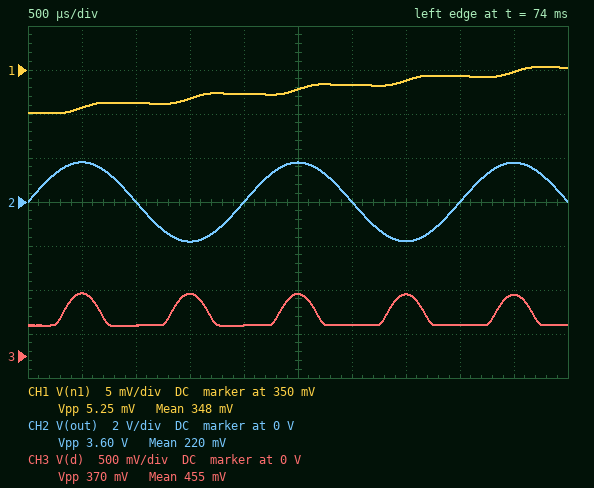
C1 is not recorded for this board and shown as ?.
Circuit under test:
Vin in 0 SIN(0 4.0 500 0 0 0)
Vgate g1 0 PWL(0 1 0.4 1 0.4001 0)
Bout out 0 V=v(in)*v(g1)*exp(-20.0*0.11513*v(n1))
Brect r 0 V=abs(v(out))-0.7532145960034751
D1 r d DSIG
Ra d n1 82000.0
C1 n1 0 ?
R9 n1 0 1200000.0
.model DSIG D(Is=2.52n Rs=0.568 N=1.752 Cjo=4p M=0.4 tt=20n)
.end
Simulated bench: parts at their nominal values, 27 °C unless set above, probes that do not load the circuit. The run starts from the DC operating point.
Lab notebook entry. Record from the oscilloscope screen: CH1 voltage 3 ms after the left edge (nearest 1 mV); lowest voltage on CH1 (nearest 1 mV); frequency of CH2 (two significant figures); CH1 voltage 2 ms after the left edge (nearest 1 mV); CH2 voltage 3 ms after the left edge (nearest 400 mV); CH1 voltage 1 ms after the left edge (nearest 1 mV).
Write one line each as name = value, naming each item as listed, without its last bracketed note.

CH1 voltage 3 ms after the left edge = 348 mV
lowest voltage on CH1 = 345 mV
frequency of CH2 = 500 Hz
CH1 voltage 2 ms after the left edge = 347 mV
CH2 voltage 3 ms after the left edge = 0 V
CH1 voltage 1 ms after the left edge = 346 mV
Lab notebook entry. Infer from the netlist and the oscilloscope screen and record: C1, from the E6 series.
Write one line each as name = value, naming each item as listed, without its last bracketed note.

C1, from the E6 series = 1 µF
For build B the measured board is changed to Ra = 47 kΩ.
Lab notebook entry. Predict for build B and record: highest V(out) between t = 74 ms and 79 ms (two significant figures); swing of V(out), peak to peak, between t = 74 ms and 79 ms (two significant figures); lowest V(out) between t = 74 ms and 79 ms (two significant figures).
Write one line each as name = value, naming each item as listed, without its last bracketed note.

highest V(out) between t = 74 ms and 79 ms = 1.7 V
swing of V(out), peak to peak, between t = 74 ms and 79 ms = 3.3 V
lowest V(out) between t = 74 ms and 79 ms = -1.7 V
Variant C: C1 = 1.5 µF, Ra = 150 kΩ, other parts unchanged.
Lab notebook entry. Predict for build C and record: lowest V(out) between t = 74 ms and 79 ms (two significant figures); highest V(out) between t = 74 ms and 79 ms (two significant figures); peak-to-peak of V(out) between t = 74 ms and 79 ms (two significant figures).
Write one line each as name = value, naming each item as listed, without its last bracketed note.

lowest V(out) between t = 74 ms and 79 ms = -2.3 V
highest V(out) between t = 74 ms and 79 ms = 2.3 V
peak-to-peak of V(out) between t = 74 ms and 79 ms = 4.6 V
